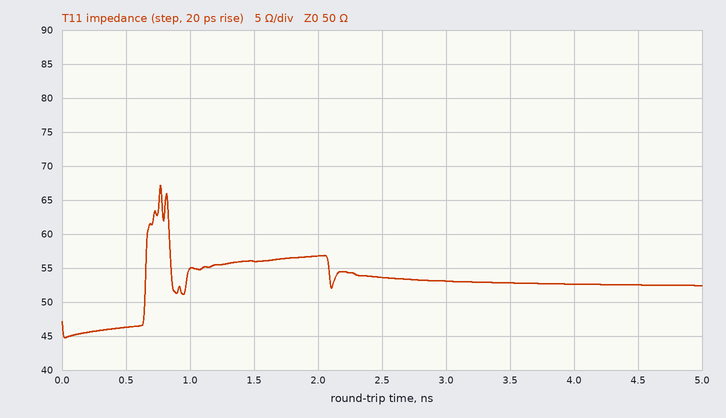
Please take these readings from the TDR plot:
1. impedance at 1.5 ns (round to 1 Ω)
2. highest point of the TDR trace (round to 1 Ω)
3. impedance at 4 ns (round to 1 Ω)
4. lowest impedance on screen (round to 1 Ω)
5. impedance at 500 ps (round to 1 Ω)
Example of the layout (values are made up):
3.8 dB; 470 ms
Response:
56 Ω; 67 Ω; 53 Ω; 45 Ω; 46 Ω
